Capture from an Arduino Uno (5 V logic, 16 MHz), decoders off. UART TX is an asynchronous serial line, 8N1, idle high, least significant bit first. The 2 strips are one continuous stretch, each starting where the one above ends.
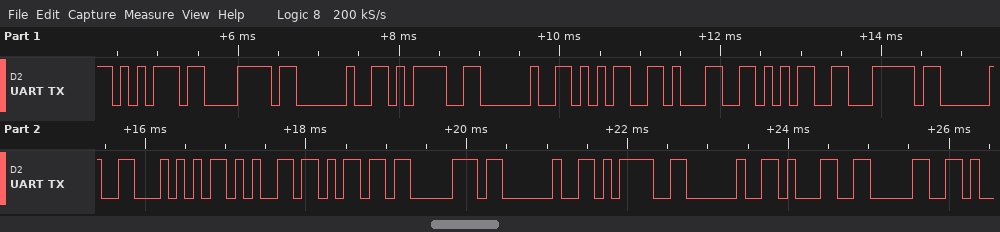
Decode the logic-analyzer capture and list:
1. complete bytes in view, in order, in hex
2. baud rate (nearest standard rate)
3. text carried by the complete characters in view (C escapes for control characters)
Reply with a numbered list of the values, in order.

1. 75 78 20 3D 20 35 31 35 7C 20 54 65 6D 70 20 3D 20 31 30
2. 9600 baud
3. "ux = 515| Temp = 10"
